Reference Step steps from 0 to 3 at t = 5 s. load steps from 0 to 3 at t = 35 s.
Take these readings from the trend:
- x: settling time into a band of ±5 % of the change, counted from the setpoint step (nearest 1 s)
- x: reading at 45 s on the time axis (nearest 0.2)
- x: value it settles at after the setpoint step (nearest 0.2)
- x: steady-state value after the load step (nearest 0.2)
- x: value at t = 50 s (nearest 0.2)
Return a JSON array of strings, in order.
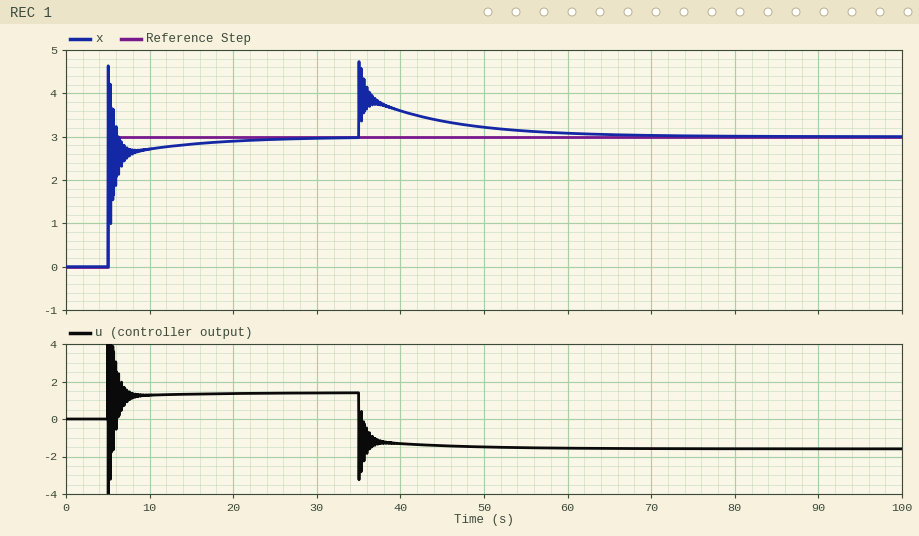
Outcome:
["11 s", "3.4", "3.0", "3.0", "3.2"]
